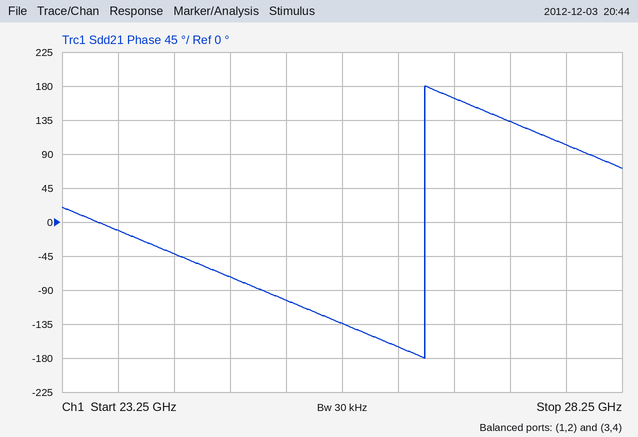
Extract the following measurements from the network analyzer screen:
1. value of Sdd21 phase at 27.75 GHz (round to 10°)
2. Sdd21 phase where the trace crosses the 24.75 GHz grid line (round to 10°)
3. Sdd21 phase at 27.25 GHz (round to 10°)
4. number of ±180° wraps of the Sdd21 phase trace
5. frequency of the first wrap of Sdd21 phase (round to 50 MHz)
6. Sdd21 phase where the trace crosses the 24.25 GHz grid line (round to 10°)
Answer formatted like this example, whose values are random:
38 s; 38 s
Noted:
100°; -70°; 130°; 1; 26.50 GHz; -40°
